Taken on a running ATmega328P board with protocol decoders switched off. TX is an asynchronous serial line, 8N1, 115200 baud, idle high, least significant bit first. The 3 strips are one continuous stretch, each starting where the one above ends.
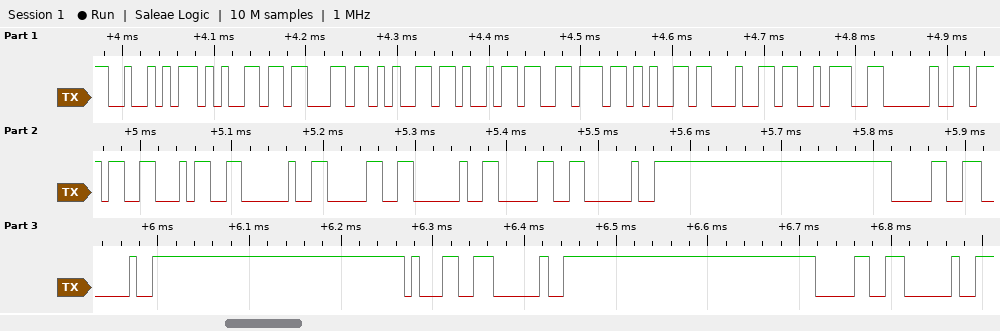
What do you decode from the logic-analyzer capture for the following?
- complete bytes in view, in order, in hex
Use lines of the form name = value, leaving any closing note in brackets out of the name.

complete bytes in view, in order, in hex = 52 65 63 65 69 76 65 64 3A 20 37 34 20 30 20 30 20 30 20 31 20 30 20
